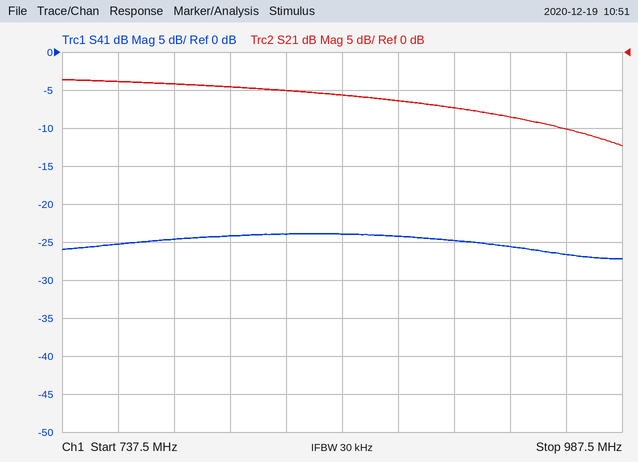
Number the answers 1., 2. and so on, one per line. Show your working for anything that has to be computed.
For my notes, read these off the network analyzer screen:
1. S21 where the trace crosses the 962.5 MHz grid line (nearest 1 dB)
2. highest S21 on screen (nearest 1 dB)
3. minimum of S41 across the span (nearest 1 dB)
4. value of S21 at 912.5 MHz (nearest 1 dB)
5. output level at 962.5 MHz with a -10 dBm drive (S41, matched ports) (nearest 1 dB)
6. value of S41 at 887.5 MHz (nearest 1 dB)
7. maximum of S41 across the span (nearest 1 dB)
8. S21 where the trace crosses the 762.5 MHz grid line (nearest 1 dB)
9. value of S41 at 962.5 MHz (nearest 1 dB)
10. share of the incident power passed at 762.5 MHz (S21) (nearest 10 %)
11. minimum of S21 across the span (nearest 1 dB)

1. -10 dB
2. -4 dB
3. -27 dB
4. -7 dB
5. -10 dBm + (-27 dB) = -37 dBm
6. -24 dB
7. -24 dB
8. -4 dB
9. -27 dB
10. 10^(-4/10) ≈ 40 %
11. -12 dB
